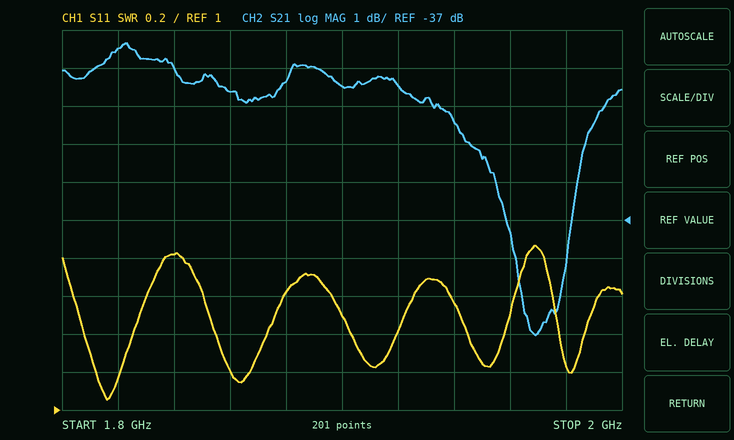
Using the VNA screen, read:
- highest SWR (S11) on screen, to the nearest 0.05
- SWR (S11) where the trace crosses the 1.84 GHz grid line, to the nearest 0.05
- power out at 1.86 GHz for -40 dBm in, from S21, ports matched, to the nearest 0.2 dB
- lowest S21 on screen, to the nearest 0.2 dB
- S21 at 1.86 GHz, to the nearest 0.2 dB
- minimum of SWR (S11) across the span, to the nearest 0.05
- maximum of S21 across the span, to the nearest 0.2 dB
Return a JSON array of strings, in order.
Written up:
["1.85", "1.80", "-73.6 dBm", "-40.0 dB", "-33.6 dB", "1.05", "-32.4 dB"]
